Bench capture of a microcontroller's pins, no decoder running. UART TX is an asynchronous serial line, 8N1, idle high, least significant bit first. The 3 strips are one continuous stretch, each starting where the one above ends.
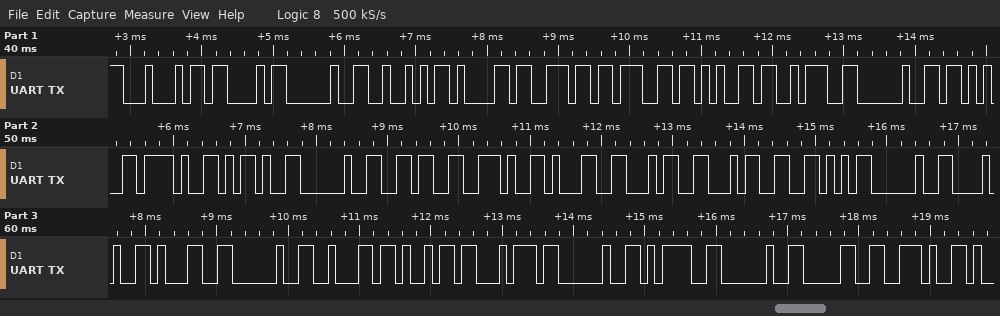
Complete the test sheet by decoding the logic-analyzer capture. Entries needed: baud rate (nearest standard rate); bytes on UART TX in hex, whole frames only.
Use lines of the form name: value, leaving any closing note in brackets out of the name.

baud rate: 9600 baud
bytes on UART TX in hex, whole frames only: 0x44 0x43 0x20 0x52 0x61 0x6E 0x67 0x65 0x3A 0x20 0x2B 0x2F 0x2D 0x20 0x36 0x2E 0x31 0x34 0x34 0x56 0x20 0x28 0x31 0x20 0x62 0x69 0x74 0x20 0x3D 0x20 0x30 0x2E
